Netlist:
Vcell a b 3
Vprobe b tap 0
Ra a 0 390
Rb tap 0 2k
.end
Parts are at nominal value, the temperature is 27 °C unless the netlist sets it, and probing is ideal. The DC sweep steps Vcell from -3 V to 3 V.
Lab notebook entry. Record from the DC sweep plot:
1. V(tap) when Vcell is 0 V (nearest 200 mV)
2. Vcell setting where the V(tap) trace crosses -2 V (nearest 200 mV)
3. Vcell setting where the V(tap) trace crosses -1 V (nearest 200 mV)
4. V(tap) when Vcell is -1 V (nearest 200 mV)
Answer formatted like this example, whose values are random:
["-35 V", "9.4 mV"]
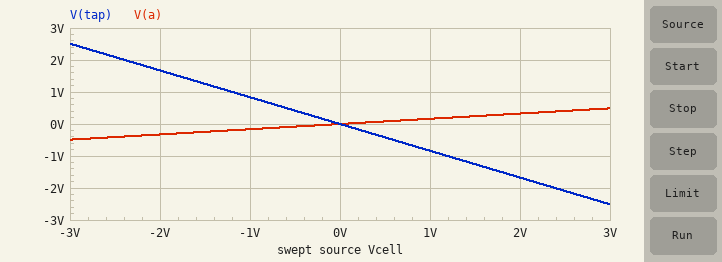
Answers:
["0 V", "2.4 V", "1.2 V", "800 mV"]
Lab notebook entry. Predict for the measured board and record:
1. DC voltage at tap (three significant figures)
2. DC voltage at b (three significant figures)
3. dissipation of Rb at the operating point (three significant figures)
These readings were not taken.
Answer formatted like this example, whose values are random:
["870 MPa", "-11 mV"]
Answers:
["-2.51 V", "-2.51 V", "3.15 mW"]
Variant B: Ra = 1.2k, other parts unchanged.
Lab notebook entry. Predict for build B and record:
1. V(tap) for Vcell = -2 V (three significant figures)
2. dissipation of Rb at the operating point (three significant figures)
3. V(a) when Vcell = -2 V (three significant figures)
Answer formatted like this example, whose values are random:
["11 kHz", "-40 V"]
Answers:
["1.25 V", "1.76 mW", "-750 mV"]
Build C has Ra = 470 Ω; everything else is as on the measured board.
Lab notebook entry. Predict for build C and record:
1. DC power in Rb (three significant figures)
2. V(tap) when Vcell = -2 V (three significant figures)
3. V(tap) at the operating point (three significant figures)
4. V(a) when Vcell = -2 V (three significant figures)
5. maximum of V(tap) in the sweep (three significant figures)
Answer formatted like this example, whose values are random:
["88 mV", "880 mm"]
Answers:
["2.95 mW", "1.62 V", "-2.43 V", "-381 mV", "2.43 V"]
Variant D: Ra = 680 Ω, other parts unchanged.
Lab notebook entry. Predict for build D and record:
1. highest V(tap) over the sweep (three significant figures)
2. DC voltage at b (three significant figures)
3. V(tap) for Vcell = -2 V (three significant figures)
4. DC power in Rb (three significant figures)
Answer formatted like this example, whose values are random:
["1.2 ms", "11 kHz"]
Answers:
["2.24 V", "-2.24 V", "1.49 V", "2.51 mW"]
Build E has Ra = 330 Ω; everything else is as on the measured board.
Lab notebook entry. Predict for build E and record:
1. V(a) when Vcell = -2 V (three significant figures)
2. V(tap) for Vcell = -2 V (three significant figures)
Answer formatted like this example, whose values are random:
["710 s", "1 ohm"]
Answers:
["-283 mV", "1.72 V"]
